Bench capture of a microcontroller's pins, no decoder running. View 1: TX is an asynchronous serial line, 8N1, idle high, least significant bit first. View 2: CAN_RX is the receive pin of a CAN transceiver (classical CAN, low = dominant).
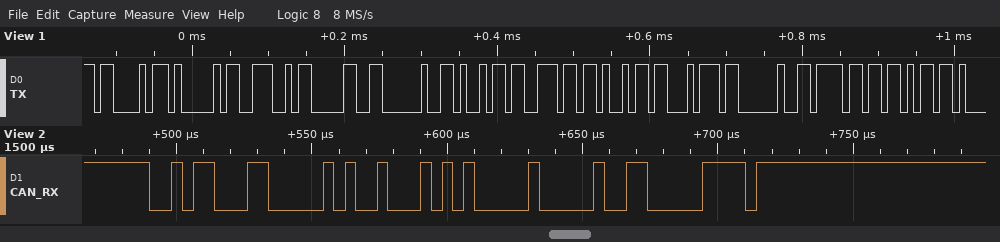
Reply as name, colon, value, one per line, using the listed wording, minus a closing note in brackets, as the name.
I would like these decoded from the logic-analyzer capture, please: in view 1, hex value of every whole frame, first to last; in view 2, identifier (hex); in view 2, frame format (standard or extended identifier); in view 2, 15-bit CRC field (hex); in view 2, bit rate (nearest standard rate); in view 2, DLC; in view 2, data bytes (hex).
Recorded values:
in view 1, hex value of every whole frame, first to last: 43 41 4E 30 20 69 6E 69 74 20 6F 6B
in view 2, identifier: 0x2C6
in view 2, frame format: standard
in view 2, 15-bit CRC field: 0x0183
in view 2, bit rate: 250 kbit/s
in view 2, DLC: 2
in view 2, data bytes: 45 40
